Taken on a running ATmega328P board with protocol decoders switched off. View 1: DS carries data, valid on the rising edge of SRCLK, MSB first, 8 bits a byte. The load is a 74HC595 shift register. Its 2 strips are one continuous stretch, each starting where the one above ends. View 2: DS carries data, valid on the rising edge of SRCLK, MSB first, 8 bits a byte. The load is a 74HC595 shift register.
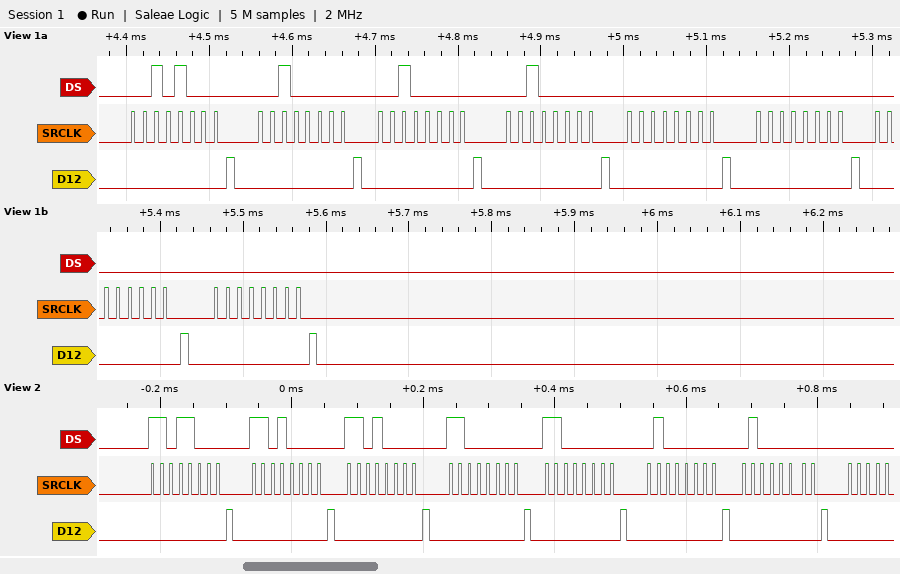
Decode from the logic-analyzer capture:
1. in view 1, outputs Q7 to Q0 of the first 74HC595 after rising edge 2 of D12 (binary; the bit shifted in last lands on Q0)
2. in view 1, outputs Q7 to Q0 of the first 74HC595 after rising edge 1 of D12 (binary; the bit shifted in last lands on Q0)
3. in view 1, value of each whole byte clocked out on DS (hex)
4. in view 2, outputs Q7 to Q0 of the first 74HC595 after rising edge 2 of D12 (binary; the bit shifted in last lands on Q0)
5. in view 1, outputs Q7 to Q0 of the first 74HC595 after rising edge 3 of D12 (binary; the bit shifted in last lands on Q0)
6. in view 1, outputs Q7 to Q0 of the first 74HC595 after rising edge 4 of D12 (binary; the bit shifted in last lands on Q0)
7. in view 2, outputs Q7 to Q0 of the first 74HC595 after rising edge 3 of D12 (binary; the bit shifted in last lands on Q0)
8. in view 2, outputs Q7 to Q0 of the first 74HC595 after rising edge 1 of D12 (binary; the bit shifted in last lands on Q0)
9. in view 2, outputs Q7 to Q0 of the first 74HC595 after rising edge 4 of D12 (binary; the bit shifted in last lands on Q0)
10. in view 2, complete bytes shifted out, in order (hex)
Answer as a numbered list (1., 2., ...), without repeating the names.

1. 00100000
2. 00101000
3. 28 20 20 20 00 00 00 00
4. 11010000
5. 00100000
6. 00100000
7. 11010000
8. 11011000
9. 11000000
10. 0xD8 0xD0 0xD0 0xC0 0xC0 0x40 0x40
